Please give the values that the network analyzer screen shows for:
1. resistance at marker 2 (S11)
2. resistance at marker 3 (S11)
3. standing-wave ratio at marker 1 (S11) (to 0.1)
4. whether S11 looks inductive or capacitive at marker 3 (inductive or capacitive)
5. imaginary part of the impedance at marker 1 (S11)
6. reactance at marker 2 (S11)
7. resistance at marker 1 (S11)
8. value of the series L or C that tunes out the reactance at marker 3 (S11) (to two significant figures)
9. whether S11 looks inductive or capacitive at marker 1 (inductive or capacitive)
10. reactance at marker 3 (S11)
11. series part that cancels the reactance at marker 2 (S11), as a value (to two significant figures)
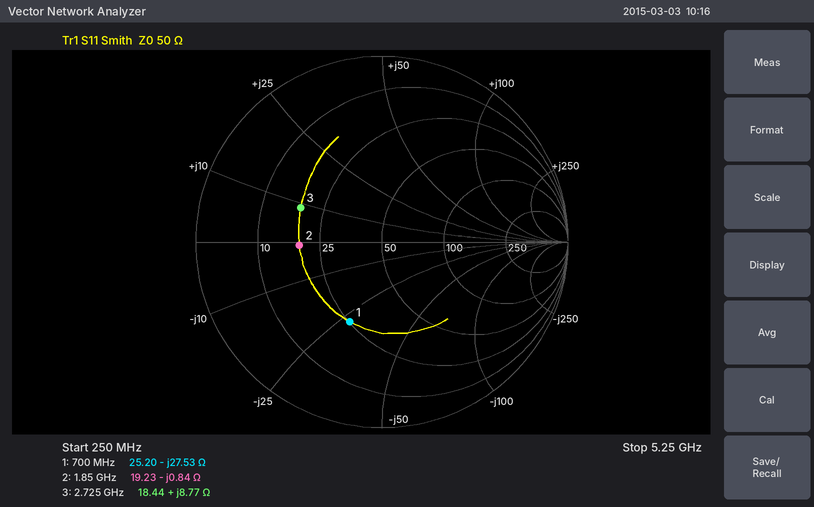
19.23 Ω
18.44 Ω
2.7
inductive
-27.53 Ω
-0.84 Ω
25.20 Ω
6.7 pF
capacitive
+8.77 Ω
72 pH
